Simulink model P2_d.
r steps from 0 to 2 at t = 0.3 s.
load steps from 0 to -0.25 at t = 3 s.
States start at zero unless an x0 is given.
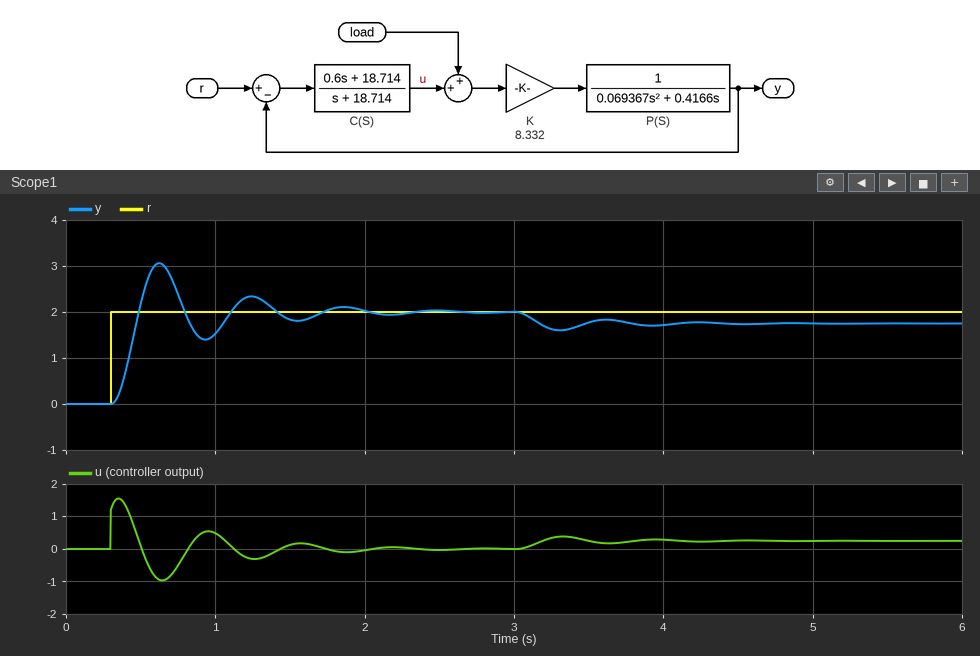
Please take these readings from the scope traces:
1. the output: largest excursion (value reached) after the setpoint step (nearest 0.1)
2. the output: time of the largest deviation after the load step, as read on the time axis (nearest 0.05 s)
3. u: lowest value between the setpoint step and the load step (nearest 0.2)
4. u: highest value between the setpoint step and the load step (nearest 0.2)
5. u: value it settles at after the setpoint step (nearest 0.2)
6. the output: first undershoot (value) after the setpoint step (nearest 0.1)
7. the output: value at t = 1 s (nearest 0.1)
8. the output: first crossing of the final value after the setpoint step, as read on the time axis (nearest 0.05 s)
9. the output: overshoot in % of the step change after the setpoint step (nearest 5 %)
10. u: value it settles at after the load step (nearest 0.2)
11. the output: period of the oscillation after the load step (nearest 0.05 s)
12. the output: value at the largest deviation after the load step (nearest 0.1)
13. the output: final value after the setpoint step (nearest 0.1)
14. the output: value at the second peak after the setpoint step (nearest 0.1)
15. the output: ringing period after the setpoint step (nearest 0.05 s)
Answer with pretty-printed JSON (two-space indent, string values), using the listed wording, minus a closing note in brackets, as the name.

{
  "the output: largest excursion (value reached) after the setpoint step": "3.1",
  "the output: time of the largest deviation after the load step, as read on the time axis": "3.30 s",
  "u: lowest value between the setpoint step and the load step": "-1.0",
  "u: highest value between the setpoint step and the load step": "1.6",
  "u: value it settles at after the setpoint step": "0.0",
  "the output: first undershoot (value) after the setpoint step": "1.4",
  "the output: value at t = 1 s": "1.5",
  "the output: first crossing of the final value after the setpoint step, as read on the time axis": "0.50 s",
  "the output: overshoot in % of the step change after the setpoint step": "55 %",
  "u: value it settles at after the load step": "0.2",
  "the output: period of the oscillation after the load step": "0.60 s",
  "the output: value at the largest deviation after the load step": "1.6",
  "the output: final value after the setpoint step": "2.0",
  "the output: value at the second peak after the setpoint step": "2.3",
  "the output: ringing period after the setpoint step": "0.60 s"
}
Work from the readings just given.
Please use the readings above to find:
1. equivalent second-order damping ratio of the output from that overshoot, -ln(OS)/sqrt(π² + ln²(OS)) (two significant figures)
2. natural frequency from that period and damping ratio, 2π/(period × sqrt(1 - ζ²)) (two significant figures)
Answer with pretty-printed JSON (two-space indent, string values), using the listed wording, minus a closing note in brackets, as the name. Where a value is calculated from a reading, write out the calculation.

{
  "equivalent second-order damping ratio of the output from that overshoot, -ln(OS)/sqrt(π² + ln²(OS))": "ln(0.55) = -0.598; 0.598 / sqrt(9.870 + 0.357) = 0.19",
  "natural frequency from that period and damping ratio, 2π/(period × sqrt(1 - ζ²))": "2π / (0.6 × sqrt(1 - 0.19²)) = 11 rad/s"
}
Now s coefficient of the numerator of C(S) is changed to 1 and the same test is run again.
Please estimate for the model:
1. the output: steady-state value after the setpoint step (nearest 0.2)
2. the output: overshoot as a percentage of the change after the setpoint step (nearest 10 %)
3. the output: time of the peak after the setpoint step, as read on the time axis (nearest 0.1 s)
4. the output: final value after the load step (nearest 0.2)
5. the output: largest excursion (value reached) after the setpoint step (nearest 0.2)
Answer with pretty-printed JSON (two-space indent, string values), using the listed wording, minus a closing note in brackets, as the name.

{
  "the output: steady-state value after the setpoint step": "2.0",
  "the output: overshoot as a percentage of the change after the setpoint step": "40 %",
  "the output: time of the peak after the setpoint step, as read on the time axis": "0.6 s",
  "the output: final value after the load step": "1.8",
  "the output: largest excursion (value reached) after the setpoint step": "2.8"
}
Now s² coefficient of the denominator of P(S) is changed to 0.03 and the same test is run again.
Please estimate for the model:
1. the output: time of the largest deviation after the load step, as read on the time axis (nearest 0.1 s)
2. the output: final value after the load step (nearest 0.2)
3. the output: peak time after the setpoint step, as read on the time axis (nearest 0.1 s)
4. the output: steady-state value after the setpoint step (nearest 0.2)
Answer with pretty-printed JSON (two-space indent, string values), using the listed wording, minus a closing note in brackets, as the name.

{
  "the output: time of the largest deviation after the load step, as read on the time axis": "3.2 s",
  "the output: final value after the load step": "1.8",
  "the output: peak time after the setpoint step, as read on the time axis": "0.5 s",
  "the output: steady-state value after the setpoint step": "2.0"
}
